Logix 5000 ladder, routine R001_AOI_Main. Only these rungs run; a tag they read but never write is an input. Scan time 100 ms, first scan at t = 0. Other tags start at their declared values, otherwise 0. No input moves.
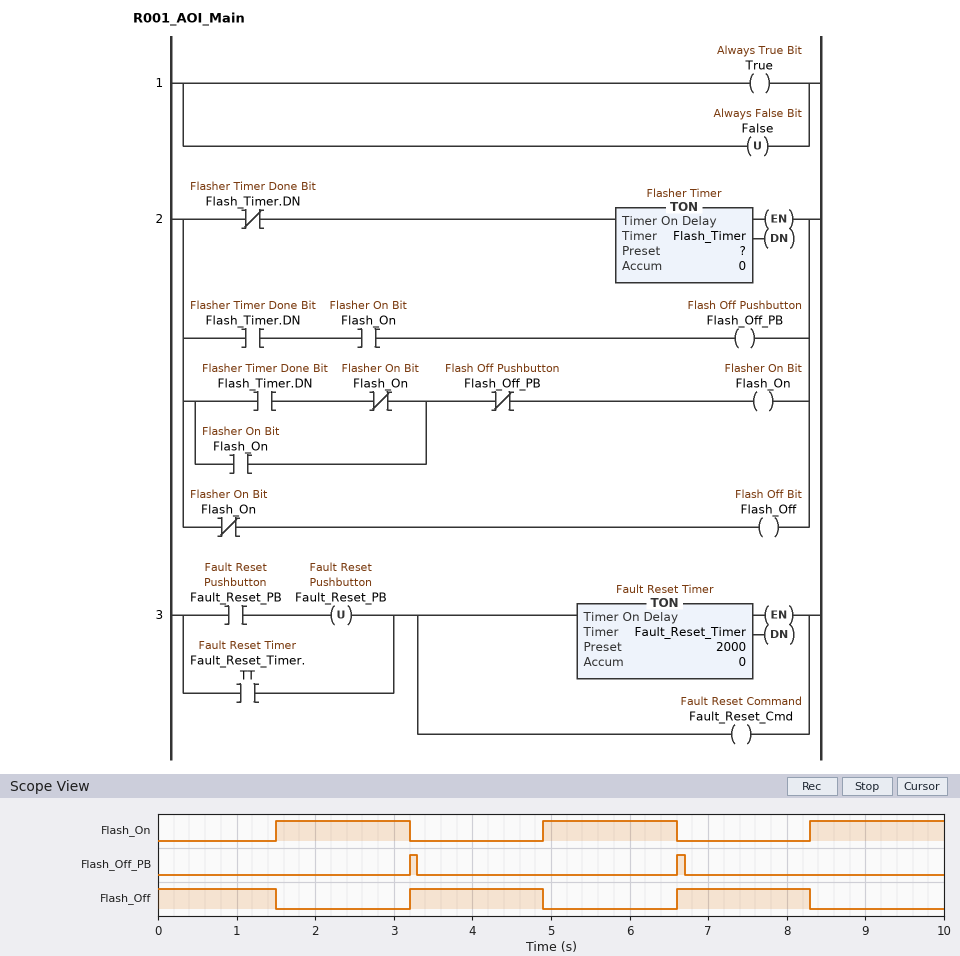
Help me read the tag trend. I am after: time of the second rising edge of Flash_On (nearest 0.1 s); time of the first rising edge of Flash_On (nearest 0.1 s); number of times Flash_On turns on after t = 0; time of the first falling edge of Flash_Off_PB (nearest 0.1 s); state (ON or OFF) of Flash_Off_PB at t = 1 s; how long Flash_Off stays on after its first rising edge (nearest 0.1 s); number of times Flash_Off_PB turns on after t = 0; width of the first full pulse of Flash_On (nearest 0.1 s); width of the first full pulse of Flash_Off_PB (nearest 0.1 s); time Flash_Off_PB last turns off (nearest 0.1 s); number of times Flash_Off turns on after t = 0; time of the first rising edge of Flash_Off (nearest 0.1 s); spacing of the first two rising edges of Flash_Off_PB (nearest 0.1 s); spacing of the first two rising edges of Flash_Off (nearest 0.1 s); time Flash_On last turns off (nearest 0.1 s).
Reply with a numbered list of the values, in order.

1. 4.9 s
2. 1.5 s
3. 3
4. 3.3 s
5. OFF
6. 1.7 s
7. 2
8. 1.7 s
9. 0.1 s
10. 6.7 s
11. 2
12. 3.2 s
13. 3.4 s
14. 3.4 s
15. 6.6 s
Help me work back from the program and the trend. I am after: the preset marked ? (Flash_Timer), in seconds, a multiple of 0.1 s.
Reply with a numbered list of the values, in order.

1. 1.5 s
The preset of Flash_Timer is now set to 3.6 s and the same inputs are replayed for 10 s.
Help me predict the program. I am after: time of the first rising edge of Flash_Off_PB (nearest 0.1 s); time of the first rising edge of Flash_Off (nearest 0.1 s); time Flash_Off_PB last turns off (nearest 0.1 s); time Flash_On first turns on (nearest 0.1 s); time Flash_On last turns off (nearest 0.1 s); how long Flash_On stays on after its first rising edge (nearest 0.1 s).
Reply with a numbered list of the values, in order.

1. 7.4 s
2. 7.4 s
3. 7.5 s
4. 3.6 s
5. 7.4 s
6. 3.8 s
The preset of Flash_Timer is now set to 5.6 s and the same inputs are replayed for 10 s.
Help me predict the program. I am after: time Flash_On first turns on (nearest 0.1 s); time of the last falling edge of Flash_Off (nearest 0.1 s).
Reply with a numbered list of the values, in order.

1. 5.6 s
2. 5.6 s
